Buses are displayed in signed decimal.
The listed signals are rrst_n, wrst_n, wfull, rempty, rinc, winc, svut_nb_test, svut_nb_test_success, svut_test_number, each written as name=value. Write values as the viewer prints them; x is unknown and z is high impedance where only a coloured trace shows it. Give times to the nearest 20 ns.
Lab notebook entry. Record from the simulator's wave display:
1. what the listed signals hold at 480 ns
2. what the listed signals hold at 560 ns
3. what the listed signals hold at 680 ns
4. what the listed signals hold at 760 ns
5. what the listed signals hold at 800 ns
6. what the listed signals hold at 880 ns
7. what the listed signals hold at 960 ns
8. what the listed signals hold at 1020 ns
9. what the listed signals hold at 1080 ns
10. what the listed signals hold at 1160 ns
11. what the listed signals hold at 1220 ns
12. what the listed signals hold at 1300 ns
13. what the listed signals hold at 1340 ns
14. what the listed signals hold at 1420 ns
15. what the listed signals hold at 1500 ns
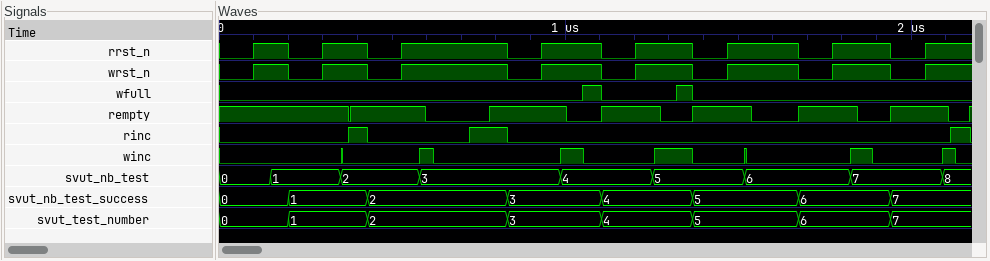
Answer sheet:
rrst_n=0, wrst_n=0, wfull=0, rempty=1, rinc=0, winc=0, svut_nb_test=2, svut_nb_test_success=2, svut_test_number=2
rrst_n=1, wrst_n=1, wfull=0, rempty=1, rinc=0, winc=0, svut_nb_test=2, svut_nb_test_success=2, svut_test_number=2
rrst_n=1, wrst_n=1, wfull=0, rempty=0, rinc=0, winc=0, svut_nb_test=3, svut_nb_test_success=2, svut_test_number=2
rrst_n=1, wrst_n=1, wfull=0, rempty=0, rinc=1, winc=0, svut_nb_test=3, svut_nb_test_success=2, svut_test_number=2
rrst_n=1, wrst_n=1, wfull=0, rempty=1, rinc=1, winc=0, svut_nb_test=3, svut_nb_test_success=2, svut_test_number=2
rrst_n=0, wrst_n=0, wfull=0, rempty=1, rinc=0, winc=0, svut_nb_test=3, svut_nb_test_success=3, svut_test_number=3
rrst_n=1, wrst_n=1, wfull=0, rempty=1, rinc=0, winc=0, svut_nb_test=3, svut_nb_test_success=3, svut_test_number=3
rrst_n=1, wrst_n=1, wfull=0, rempty=0, rinc=0, winc=1, svut_nb_test=4, svut_nb_test_success=3, svut_test_number=3
rrst_n=1, wrst_n=1, wfull=1, rempty=0, rinc=0, winc=0, svut_nb_test=4, svut_nb_test_success=3, svut_test_number=3
rrst_n=0, wrst_n=0, wfull=0, rempty=1, rinc=0, winc=0, svut_nb_test=4, svut_nb_test_success=4, svut_test_number=4
rrst_n=1, wrst_n=1, wfull=0, rempty=1, rinc=0, winc=0, svut_nb_test=4, svut_nb_test_success=4, svut_test_number=4
rrst_n=1, wrst_n=1, wfull=0, rempty=0, rinc=0, winc=1, svut_nb_test=5, svut_nb_test_success=4, svut_test_number=4
rrst_n=1, wrst_n=1, wfull=1, rempty=0, rinc=0, winc=1, svut_nb_test=5, svut_nb_test_success=4, svut_test_number=4
rrst_n=0, wrst_n=0, wfull=0, rempty=1, rinc=0, winc=0, svut_nb_test=5, svut_nb_test_success=5, svut_test_number=5
rrst_n=1, wrst_n=1, wfull=0, rempty=1, rinc=0, winc=0, svut_nb_test=5, svut_nb_test_success=5, svut_test_number=5
